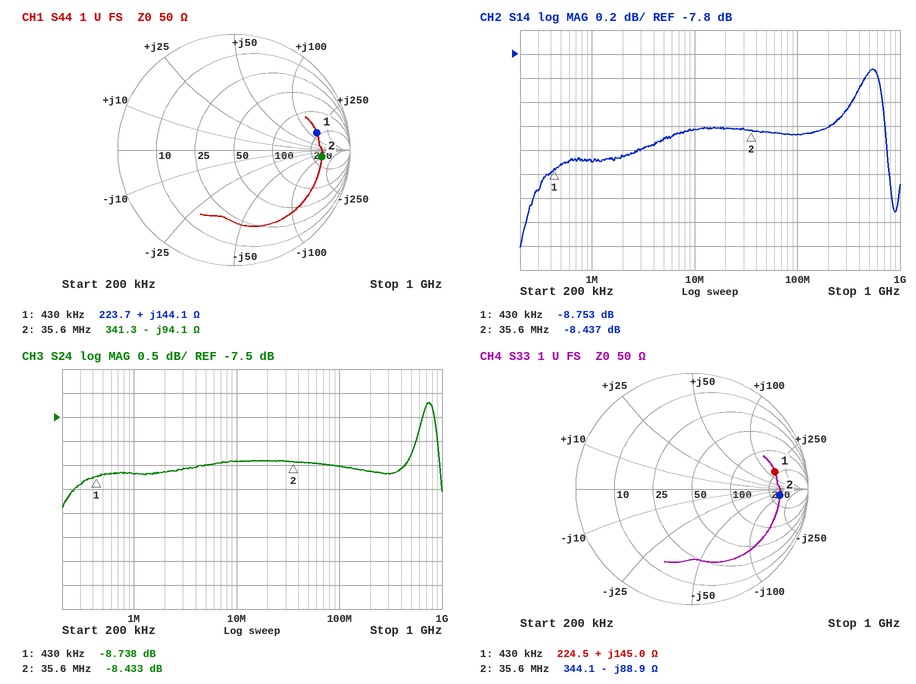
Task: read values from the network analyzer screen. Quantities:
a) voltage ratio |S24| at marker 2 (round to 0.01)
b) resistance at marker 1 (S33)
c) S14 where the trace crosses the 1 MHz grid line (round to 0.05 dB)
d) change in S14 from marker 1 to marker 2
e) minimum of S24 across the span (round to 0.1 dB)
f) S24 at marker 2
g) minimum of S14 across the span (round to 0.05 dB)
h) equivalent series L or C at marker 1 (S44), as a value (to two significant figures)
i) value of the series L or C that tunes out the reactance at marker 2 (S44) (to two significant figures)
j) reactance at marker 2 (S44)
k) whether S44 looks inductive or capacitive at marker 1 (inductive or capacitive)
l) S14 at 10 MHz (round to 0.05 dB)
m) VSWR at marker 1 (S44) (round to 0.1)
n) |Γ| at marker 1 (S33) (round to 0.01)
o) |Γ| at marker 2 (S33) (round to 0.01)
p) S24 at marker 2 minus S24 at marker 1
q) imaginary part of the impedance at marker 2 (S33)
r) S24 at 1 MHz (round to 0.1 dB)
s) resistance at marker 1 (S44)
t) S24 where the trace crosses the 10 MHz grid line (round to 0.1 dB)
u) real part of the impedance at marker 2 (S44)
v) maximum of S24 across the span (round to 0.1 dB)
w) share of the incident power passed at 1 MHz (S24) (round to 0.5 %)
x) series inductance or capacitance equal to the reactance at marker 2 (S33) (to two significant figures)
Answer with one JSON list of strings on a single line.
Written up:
["0.38", "224.5 Ω", "-8.70 dB", "0.316 dB", "-9.4 dB", "-8.433 dB", "-9.40 dB", "53 µH", "420 nH", "-94.1 Ω", "inductive", "-8.45 dB", "6.4", "0.73", "0.76", "0.305 dB", "-88.9 Ω", "-8.7 dB", "223.7 Ω", "-8.4 dB", "341.3 Ω", "-7.2 dB", "13.5 %", "50 pF"]
